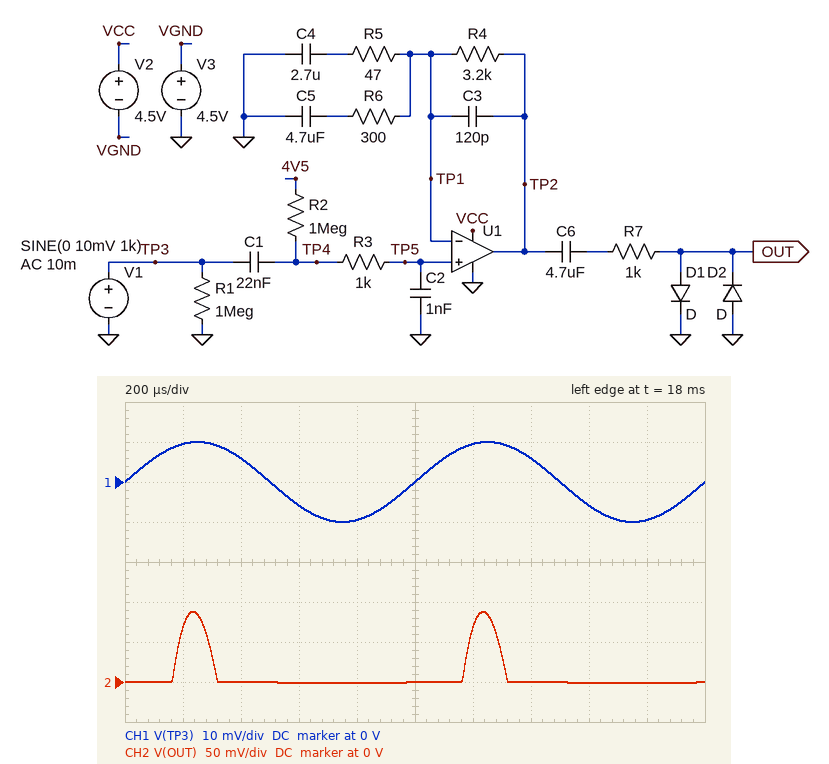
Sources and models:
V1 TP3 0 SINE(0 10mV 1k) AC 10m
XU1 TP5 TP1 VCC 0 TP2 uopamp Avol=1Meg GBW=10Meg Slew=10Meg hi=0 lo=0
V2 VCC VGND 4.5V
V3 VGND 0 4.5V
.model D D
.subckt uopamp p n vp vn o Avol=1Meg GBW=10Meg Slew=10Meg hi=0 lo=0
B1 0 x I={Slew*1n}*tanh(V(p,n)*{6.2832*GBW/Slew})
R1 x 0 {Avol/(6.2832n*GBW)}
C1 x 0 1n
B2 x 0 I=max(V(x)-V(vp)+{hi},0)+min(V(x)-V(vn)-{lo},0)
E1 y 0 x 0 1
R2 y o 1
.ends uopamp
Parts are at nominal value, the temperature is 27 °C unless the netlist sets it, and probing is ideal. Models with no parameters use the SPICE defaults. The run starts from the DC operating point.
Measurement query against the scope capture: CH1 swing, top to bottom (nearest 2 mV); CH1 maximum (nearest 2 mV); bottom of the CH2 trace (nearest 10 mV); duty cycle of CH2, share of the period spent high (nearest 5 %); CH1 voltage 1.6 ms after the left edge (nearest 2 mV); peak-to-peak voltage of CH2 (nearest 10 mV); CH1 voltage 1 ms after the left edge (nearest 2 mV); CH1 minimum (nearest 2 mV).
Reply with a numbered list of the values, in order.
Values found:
1. 20 mV
2. 10 mV
3. 0 V
4. 10 %
5. -6 mV
6. 90 mV
7. 0 V
8. -10 mV
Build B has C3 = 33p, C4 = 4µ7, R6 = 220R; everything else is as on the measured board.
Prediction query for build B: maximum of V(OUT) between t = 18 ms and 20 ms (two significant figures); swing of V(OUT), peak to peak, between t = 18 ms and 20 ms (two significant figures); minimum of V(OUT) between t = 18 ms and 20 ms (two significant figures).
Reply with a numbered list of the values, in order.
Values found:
1. 90 mV
2. 91 mV
3. -1.2 mV
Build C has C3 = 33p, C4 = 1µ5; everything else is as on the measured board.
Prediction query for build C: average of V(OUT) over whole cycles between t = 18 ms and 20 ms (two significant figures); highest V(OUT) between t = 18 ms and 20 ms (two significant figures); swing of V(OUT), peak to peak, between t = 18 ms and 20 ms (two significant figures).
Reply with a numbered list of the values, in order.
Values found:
1. 8.4 mV
2. 85 mV
3. 86 mV
